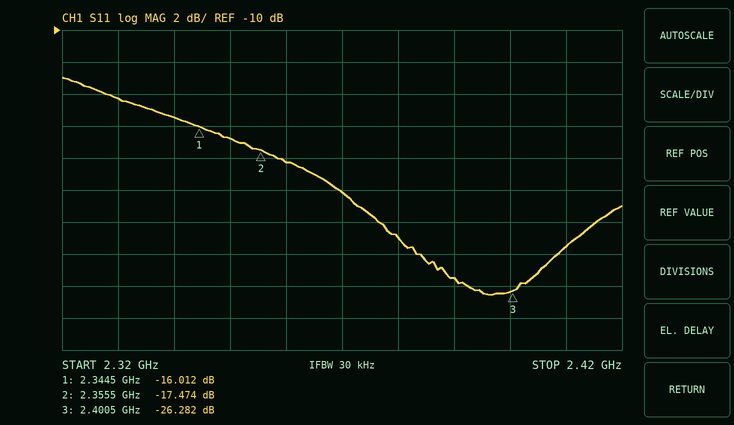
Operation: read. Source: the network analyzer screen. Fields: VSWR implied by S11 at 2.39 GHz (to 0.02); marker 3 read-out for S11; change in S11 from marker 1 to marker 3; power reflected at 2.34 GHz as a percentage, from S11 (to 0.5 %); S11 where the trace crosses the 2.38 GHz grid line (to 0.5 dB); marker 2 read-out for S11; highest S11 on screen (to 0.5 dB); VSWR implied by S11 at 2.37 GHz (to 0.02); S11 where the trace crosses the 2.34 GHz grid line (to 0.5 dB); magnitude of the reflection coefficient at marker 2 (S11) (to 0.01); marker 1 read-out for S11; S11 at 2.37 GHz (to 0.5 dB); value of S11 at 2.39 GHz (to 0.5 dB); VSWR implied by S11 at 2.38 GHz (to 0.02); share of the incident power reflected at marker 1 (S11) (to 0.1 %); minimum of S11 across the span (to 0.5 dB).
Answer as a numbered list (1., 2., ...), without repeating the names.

1. 1.12
2. -26.282 dB
3. -10.270 dB
4. 3.0 %
5. -23.0 dB
6. -17.474 dB
7. -13.0 dB
8. 1.22
9. -15.5 dB
10. 0.13
11. -16.012 dB
12. -20.0 dB
13. -25.5 dB
14. 1.16
15. 2.5 %
16. -26.5 dB
